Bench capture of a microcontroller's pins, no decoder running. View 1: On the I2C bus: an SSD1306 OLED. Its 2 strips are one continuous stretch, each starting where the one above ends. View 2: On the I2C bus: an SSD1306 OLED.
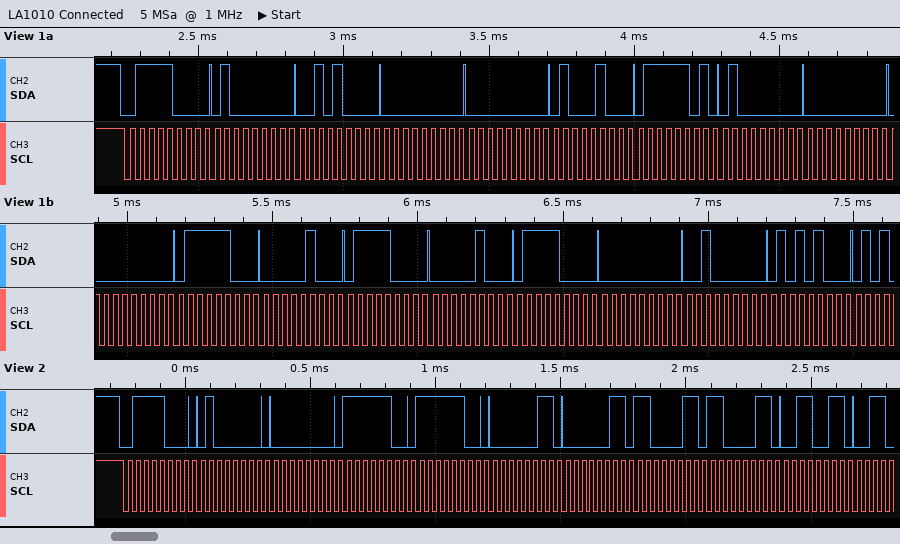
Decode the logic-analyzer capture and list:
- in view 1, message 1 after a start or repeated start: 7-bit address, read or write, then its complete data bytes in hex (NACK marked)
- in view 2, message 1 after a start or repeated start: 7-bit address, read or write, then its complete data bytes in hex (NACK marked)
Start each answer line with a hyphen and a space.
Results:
- 0x3C write: 40 28 00 00 44 7D 40 00 00 7C 04 78 04 78 00 20 54
- 0x3C write: 40 00 FC FC 03 03 C3 C3 33
